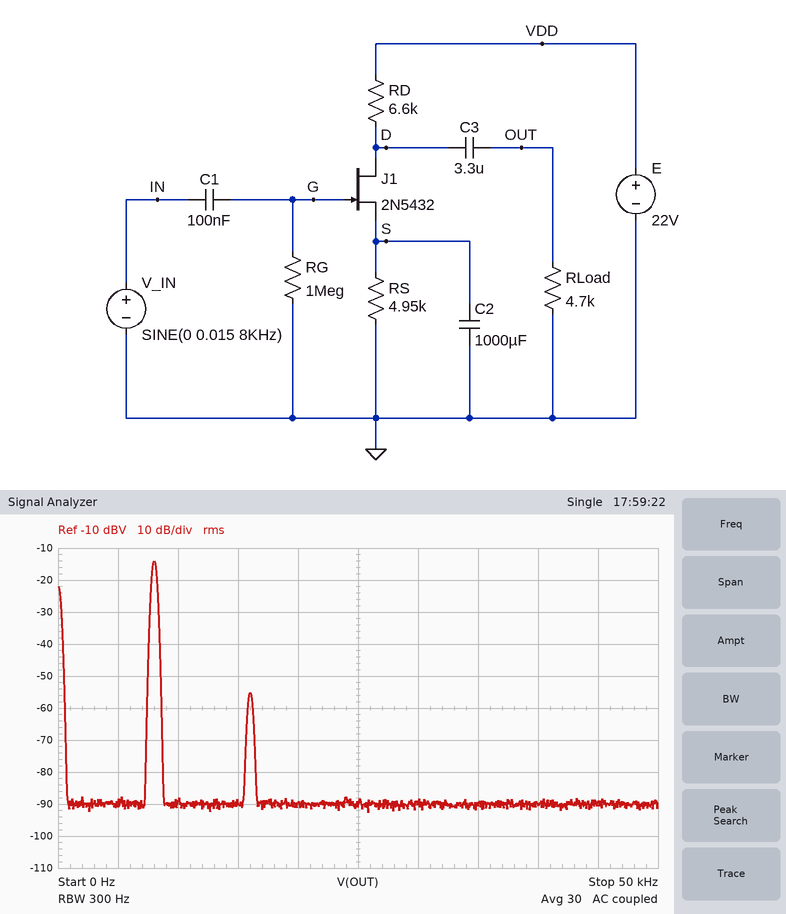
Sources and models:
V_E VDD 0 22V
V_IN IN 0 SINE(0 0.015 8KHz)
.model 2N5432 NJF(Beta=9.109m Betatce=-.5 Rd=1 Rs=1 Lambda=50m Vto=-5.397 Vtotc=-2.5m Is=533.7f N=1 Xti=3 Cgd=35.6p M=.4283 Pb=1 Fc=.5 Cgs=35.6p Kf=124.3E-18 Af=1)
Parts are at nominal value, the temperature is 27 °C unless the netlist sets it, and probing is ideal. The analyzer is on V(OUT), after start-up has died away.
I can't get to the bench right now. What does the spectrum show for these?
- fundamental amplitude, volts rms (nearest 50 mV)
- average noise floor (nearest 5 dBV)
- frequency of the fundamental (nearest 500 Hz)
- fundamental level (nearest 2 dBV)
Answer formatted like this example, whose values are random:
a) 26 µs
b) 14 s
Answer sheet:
a) 200 mV
b) -90 dBV
c) 8.0 kHz
d) -14 dBV
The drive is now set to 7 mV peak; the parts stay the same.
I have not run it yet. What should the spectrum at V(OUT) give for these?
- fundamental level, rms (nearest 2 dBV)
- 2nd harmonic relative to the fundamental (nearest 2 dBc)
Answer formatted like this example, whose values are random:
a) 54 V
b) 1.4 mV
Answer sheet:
a) -20 dBV
b) -48 dBc
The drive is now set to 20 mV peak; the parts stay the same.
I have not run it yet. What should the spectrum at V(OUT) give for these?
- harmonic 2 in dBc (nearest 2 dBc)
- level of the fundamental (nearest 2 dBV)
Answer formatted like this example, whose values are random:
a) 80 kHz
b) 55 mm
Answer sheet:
a) -38 dBc
b) -12 dBV
